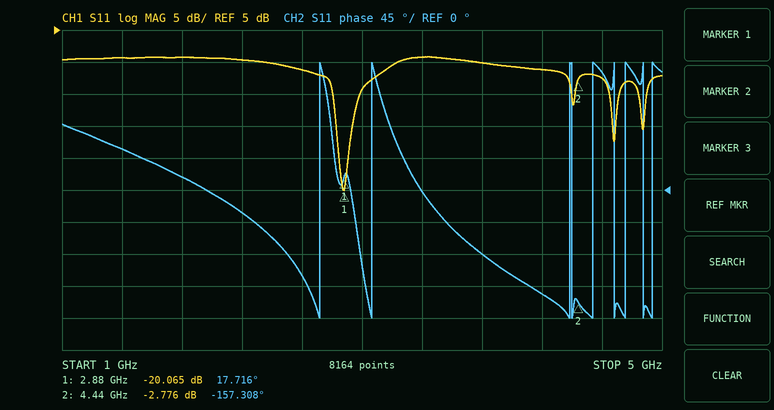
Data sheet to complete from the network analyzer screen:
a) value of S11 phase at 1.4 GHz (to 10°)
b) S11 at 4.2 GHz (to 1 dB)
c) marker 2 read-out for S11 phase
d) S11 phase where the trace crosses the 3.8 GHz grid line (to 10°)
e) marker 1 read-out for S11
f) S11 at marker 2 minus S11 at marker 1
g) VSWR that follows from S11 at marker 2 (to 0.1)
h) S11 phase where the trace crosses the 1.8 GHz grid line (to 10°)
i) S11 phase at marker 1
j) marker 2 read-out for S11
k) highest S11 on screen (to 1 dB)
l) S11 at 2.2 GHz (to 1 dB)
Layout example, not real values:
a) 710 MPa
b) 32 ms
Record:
a) 60°
b) -1 dB
c) -157.308°
d) -90°
e) -20.065 dB
f) 17.289 dB
g) 6.3
h) 20°
i) 17.716°
j) -2.776 dB
k) 1 dB
l) 0 dB
